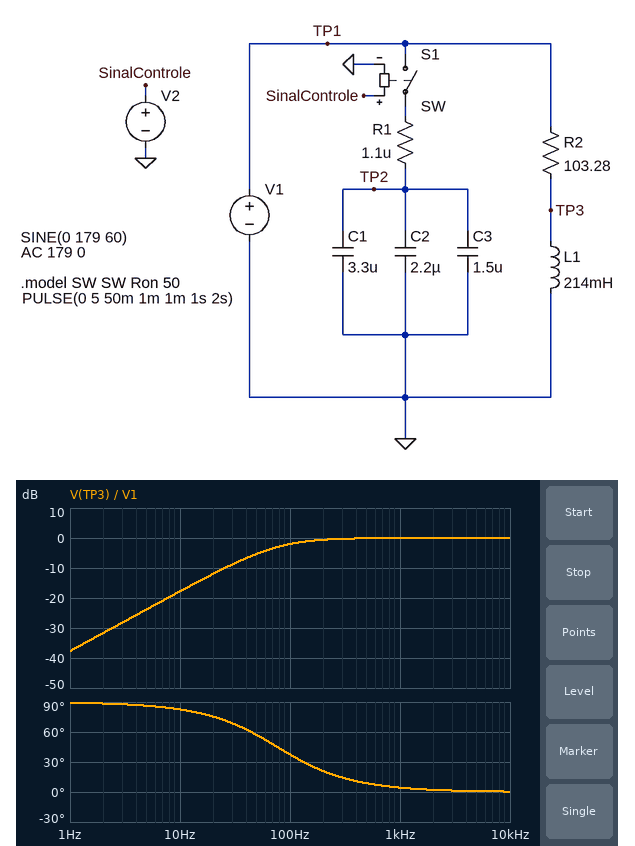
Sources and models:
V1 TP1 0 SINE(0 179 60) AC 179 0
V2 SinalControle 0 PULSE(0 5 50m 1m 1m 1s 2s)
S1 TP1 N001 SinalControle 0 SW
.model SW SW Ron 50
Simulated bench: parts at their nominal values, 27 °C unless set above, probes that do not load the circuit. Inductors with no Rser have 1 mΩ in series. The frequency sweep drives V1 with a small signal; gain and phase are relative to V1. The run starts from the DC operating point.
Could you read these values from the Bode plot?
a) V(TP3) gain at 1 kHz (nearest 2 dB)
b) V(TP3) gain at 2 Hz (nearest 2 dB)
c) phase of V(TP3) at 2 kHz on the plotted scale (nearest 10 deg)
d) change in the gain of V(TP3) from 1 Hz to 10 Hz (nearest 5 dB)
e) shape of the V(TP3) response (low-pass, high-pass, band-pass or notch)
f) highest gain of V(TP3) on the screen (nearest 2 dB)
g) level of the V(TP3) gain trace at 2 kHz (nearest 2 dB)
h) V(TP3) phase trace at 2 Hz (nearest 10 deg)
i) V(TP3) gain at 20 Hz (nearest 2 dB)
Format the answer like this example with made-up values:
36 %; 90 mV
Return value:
0 dB; -32 dB; 0 deg; 20 dB; high-pass; 0 dB; 0 dB; 90 deg; -12 dB
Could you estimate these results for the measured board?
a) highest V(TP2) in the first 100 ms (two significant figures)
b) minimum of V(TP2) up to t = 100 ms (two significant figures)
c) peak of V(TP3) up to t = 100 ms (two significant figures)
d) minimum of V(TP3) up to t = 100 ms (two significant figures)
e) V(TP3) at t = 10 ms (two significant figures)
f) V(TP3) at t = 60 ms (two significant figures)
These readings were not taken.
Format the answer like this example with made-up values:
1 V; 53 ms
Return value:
180 V; -180 V; 110 V; -110 V; -110 V; -110 V
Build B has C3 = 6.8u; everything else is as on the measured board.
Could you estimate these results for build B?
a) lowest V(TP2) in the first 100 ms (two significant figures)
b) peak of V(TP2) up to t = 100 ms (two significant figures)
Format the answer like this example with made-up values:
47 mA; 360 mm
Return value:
-170 V; 170 V
